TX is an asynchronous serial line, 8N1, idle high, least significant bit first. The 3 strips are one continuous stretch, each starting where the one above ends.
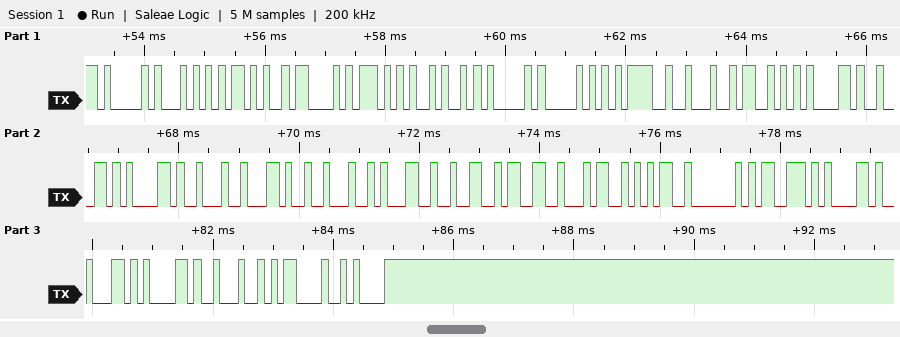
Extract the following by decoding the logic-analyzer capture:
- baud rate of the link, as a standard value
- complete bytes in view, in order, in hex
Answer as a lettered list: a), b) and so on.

a) 9600 baud
b) 41 54 2B 43 57 4A 41 50 3D 22 53 61 62 61 22 2C 22 31 32 33 34 35 40 73 61 62 61 22 0D 0A
